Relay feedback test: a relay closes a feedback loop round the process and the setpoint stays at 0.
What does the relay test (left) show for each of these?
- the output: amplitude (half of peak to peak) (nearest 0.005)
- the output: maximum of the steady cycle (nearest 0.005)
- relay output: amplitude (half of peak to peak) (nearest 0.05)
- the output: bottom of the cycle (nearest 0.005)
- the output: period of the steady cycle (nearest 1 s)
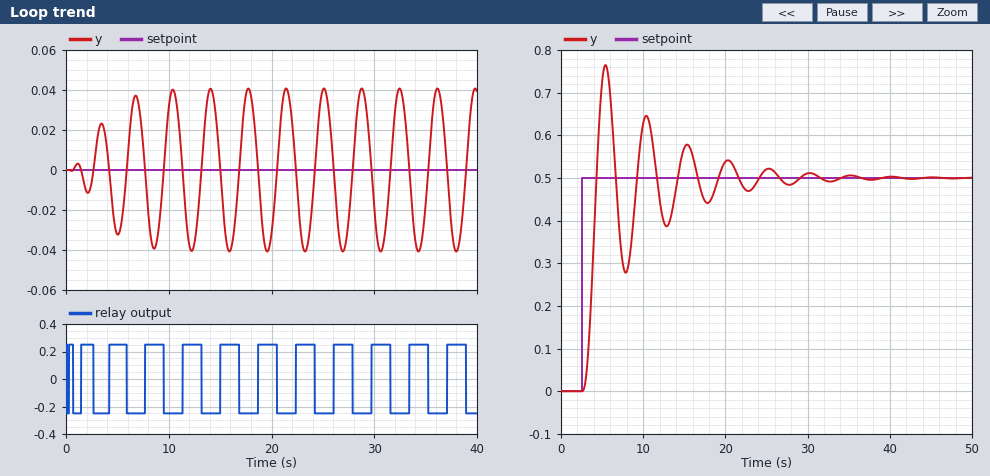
0.040
0.040
0.25
-0.040
4 s
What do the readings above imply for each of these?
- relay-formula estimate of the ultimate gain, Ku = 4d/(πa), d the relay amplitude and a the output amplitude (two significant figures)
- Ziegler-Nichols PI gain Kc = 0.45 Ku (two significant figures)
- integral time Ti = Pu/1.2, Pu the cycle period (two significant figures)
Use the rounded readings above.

8.0
3.6
3.3 s
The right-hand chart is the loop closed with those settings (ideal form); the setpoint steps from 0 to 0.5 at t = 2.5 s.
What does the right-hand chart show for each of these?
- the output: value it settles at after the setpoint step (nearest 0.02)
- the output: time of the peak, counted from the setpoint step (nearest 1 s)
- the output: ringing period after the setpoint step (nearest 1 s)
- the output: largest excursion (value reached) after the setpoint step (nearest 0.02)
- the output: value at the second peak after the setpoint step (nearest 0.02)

0.50
3 s
5 s
0.76
0.64
